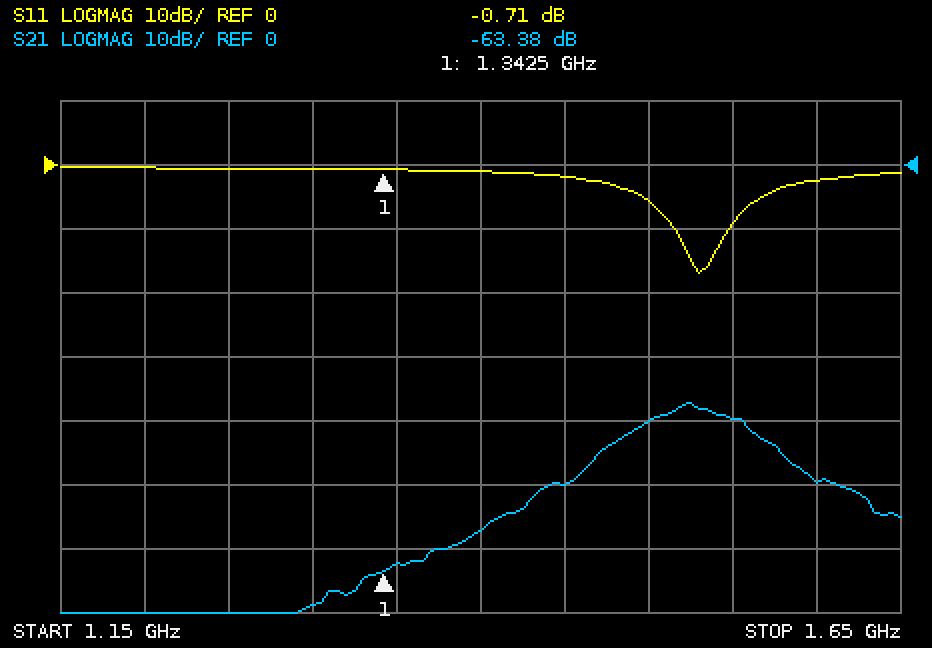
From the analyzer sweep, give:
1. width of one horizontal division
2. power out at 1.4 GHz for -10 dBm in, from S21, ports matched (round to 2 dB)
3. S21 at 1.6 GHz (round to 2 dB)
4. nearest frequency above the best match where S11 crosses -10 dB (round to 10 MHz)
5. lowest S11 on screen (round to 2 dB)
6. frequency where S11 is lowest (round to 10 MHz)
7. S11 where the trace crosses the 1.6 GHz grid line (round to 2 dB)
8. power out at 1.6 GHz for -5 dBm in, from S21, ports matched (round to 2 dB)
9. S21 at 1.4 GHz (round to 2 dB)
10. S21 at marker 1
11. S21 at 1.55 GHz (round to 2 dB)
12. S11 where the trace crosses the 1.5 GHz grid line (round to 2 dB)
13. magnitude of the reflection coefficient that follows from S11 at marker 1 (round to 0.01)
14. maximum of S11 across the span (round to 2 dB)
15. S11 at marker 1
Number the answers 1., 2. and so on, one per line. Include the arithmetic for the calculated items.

1. 50 MHz
2. -10 dBm + (-58 dB) = -68 dBm
3. -50 dB
4. 1.55 GHz
5. -16 dB
6. 1.53 GHz
7. -2 dB
8. -5 dBm + (-50 dB) = -54 dBm
9. -58 dB
10. -63.38 dB
11. -40 dB
12. -6 dB
13. 10^(-0.71/20) ≈ 0.92
14. 0 dB
15. -0.71 dB
